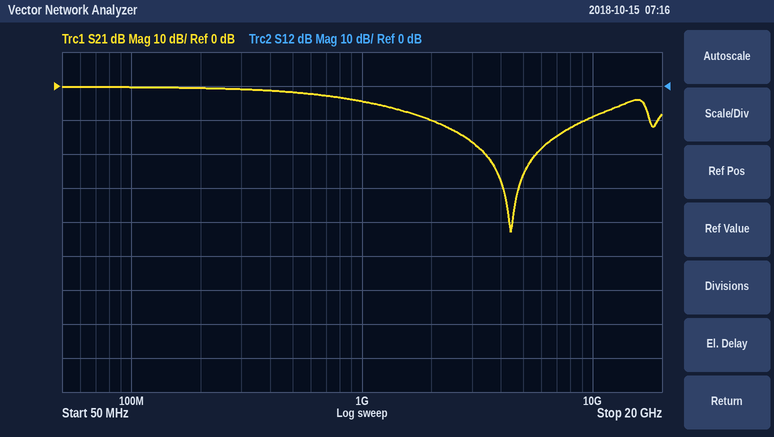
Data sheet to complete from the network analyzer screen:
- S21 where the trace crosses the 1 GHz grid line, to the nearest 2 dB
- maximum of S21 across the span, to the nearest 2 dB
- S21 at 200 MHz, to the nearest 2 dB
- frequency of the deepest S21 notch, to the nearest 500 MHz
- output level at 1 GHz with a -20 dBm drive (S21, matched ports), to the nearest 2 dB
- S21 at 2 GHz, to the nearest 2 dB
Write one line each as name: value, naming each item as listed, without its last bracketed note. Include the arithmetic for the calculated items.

S21 where the trace crosses the 1 GHz grid line, to the nearest 2 dB: -4 dB
maximum of S21 across the span, to the nearest 2 dB: 0 dB
S21 at 200 MHz, to the nearest 2 dB: 0 dB
frequency of the deepest S21 notch, to the nearest 500 MHz: 4.5 GHz
output level at 1 GHz with a -20 dBm drive (S21, matched ports), to the nearest 2 dB: -20 dBm + (-4 dB) = -24 dBm
S21 at 2 GHz, to the nearest 2 dB: -10 dB
